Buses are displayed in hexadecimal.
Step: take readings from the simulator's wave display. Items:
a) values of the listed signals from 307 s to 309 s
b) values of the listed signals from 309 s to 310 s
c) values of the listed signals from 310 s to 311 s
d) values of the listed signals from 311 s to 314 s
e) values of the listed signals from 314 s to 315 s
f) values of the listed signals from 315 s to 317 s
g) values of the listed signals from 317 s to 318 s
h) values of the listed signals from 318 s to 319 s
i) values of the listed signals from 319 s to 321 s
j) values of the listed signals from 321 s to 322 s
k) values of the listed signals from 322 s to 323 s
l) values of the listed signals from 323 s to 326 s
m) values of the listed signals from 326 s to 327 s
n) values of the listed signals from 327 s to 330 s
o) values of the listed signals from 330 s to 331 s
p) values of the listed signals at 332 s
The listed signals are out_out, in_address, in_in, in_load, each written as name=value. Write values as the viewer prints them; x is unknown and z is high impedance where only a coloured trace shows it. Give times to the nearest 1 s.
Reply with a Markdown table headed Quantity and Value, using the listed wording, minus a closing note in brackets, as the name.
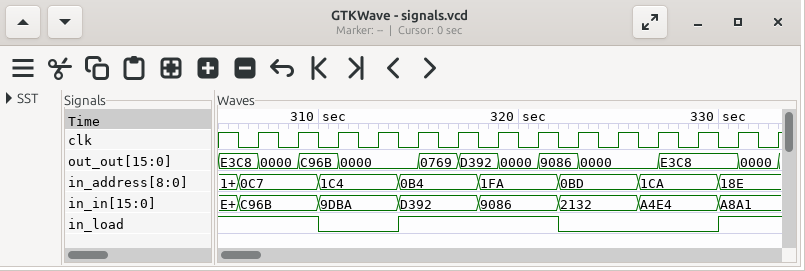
| Quantity | Value |
|---|---|
| values of the listed signals from 307 s to 309 s | out_out=0000, in_address=0C7, in_in=C96B, in_load=1 |
| values of the listed signals from 309 s to 310 s | out_out=C96B, in_address=0C7, in_in=C96B, in_load=1 |
| values of the listed signals from 310 s to 311 s | out_out=C96B, in_address=1C4, in_in=9DBA, in_load=0 |
| values of the listed signals from 311 s to 314 s | out_out=0000, in_address=1C4, in_in=9DBA, in_load=0 |
| values of the listed signals from 314 s to 315 s | out_out=0000, in_address=0B4, in_in=D392, in_load=1 |
| values of the listed signals from 315 s to 317 s | out_out=0769, in_address=0B4, in_in=D392, in_load=1 |
| values of the listed signals from 317 s to 318 s | out_out=D392, in_address=0B4, in_in=D392, in_load=1 |
| values of the listed signals from 318 s to 319 s | out_out=D392, in_address=1FA, in_in=9086, in_load=1 |
| values of the listed signals from 319 s to 321 s | out_out=0000, in_address=1FA, in_in=9086, in_load=1 |
| values of the listed signals from 321 s to 322 s | out_out=9086, in_address=1FA, in_in=9086, in_load=1 |
| values of the listed signals from 322 s to 323 s | out_out=9086, in_address=0BD, in_in=2132, in_load=0 |
| values of the listed signals from 323 s to 326 s | out_out=0000, in_address=0BD, in_in=2132, in_load=0 |
| values of the listed signals from 326 s to 327 s | out_out=0000, in_address=1CA, in_in=A4E4, in_load=0 |
| values of the listed signals from 327 s to 330 s | out_out=E3C8, in_address=1CA, in_in=A4E4, in_load=0 |
| values of the listed signals from 330 s to 331 s | out_out=E3C8, in_address=18E, in_in=A8A1, in_load=1 |
| values of the listed signals at 332 s | out_out=0000, in_address=18E, in_in=A8A1, in_load=1 |
